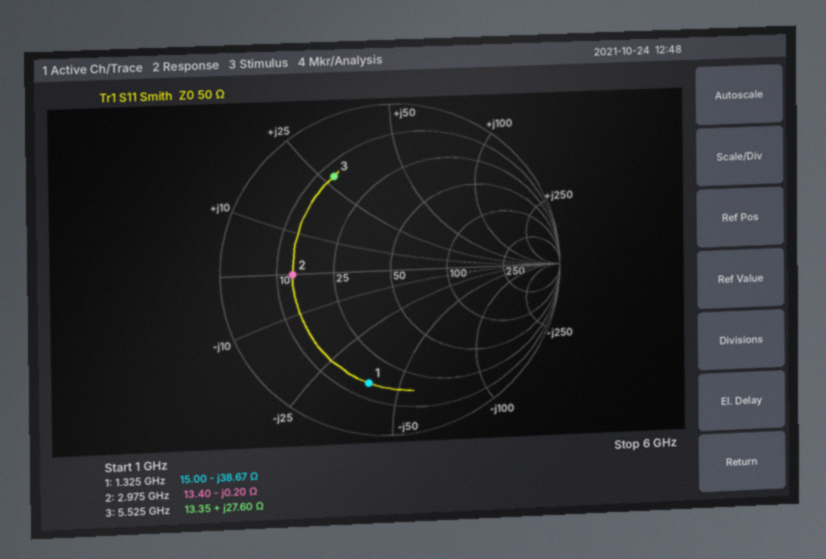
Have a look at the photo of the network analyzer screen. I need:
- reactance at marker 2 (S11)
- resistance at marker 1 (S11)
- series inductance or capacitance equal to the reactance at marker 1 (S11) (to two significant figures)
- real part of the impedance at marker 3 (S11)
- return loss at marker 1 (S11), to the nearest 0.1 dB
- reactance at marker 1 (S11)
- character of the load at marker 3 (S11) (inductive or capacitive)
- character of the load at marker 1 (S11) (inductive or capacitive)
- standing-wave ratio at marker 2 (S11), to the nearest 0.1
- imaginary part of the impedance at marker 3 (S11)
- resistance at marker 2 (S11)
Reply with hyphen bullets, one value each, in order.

- -0.20 Ω
- 15.00 Ω
- 3.1 pF
- 13.35 Ω
- 3.2 dB
- -38.67 Ω
- inductive
- capacitive
- 3.7
- +27.60 Ω
- 13.40 Ω
